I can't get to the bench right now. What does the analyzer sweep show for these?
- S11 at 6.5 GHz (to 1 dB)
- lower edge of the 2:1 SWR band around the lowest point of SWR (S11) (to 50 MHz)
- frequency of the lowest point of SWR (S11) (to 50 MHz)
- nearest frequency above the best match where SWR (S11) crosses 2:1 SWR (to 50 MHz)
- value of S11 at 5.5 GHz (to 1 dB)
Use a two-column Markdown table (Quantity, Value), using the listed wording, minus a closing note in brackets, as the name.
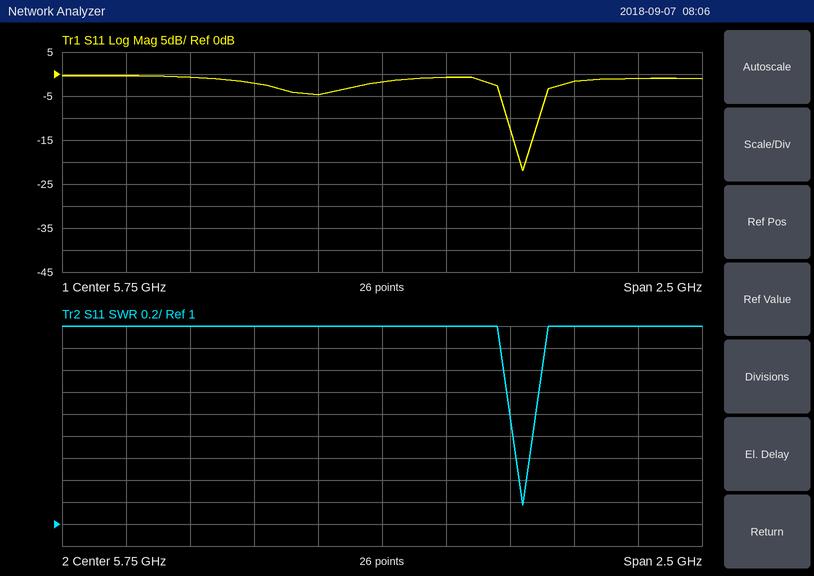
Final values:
| Quantity | Value |
|---|---|
| S11 at 6.5 GHz | -2 dB |
| lower edge of the 2:1 SWR band around the lowest point of SWR (S11) | 6.25 GHz |
| frequency of the lowest point of SWR (S11) | 6.30 GHz |
| nearest frequency above the best match where SWR (S11) crosses 2:1 SWR | 6.35 GHz |
| value of S11 at 5.5 GHz | -5 dB |
